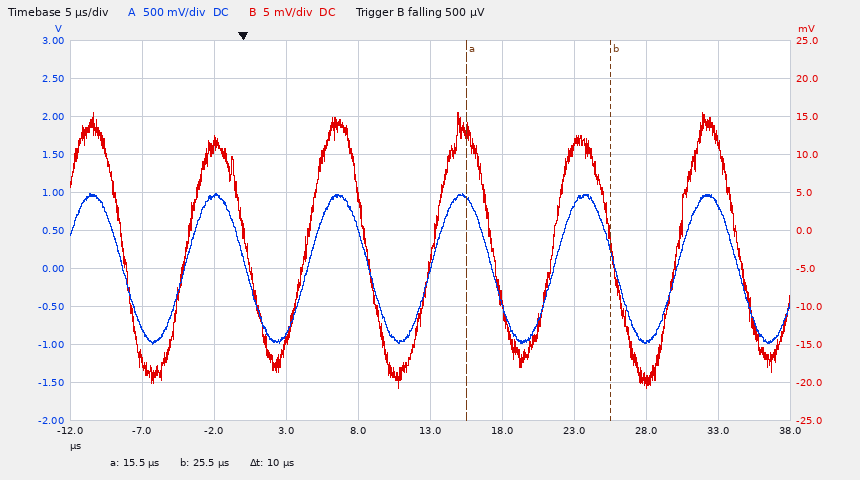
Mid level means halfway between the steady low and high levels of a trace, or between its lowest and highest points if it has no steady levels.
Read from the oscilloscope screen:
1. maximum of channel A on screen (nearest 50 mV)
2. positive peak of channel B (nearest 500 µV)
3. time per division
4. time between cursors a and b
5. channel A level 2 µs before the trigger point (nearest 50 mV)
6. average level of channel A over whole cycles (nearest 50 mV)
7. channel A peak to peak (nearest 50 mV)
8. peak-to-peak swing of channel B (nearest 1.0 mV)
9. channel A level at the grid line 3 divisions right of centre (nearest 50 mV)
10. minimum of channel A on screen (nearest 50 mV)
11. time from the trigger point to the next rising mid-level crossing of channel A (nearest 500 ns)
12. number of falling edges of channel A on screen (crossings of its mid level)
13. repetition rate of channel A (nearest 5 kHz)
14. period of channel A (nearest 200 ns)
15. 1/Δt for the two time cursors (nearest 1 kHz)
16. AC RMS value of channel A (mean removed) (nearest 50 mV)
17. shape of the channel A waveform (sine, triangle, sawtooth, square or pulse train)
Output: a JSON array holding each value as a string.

["1.00 V", "15.5 mV", "5 µs", "10 µs", "950 mV", "0 mV", "2.00 V", "36.0 mV", "-950 mV", "-1.00 V", "4.5 µs", "6", "115 kHz", "8.6 µs", "100 kHz", "700 mV", "sine"]
